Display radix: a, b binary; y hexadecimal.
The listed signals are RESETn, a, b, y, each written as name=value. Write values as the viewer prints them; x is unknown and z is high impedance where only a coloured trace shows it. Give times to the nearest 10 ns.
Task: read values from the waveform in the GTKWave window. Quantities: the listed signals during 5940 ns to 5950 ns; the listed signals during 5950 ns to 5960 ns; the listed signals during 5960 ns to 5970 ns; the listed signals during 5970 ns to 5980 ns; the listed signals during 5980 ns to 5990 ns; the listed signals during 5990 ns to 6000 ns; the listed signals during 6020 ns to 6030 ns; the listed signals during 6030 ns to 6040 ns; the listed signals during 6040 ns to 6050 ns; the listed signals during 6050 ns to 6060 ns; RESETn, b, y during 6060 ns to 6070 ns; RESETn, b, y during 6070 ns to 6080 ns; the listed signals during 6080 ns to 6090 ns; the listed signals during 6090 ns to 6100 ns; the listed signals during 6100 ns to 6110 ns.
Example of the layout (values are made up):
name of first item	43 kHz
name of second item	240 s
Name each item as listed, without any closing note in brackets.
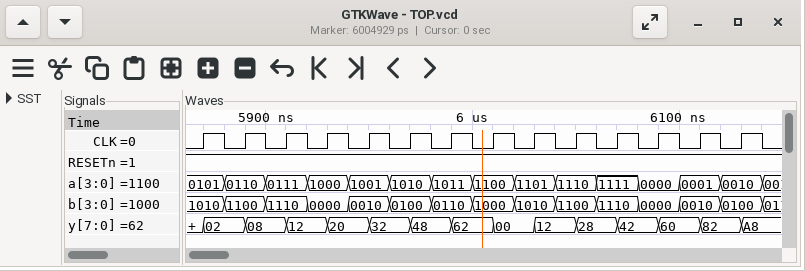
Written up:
the listed signals during 5940 ns to 5950 ns	RESETn=1, a=1001, b=0010, y=20
the listed signals during 5950 ns to 5960 ns	RESETn=1, a=1001, b=0010, y=32
the listed signals during 5960 ns to 5970 ns	RESETn=1, a=1010, b=0100, y=32
the listed signals during 5970 ns to 5980 ns	RESETn=1, a=1010, b=0100, y=48
the listed signals during 5980 ns to 5990 ns	RESETn=1, a=1011, b=0110, y=48
the listed signals during 5990 ns to 6000 ns	RESETn=1, a=1011, b=0110, y=62
the listed signals during 6020 ns to 6030 ns	RESETn=1, a=1101, b=1010, y=00
the listed signals during 6030 ns to 6040 ns	RESETn=1, a=1101, b=1010, y=12
the listed signals during 6040 ns to 6050 ns	RESETn=1, a=1110, b=1100, y=12
the listed signals during 6050 ns to 6060 ns	RESETn=1, a=1110, b=1100, y=28
RESETn, b, y during 6060 ns to 6070 ns	RESETn=1, b=1110, y=28
RESETn, b, y during 6070 ns to 6080 ns	RESETn=1, b=1110, y=42
the listed signals during 6080 ns to 6090 ns	RESETn=1, a=0000, b=0000, y=42
the listed signals during 6090 ns to 6100 ns	RESETn=1, a=0000, b=0000, y=60
the listed signals during 6100 ns to 6110 ns	RESETn=1, a=0001, b=0010, y=60
